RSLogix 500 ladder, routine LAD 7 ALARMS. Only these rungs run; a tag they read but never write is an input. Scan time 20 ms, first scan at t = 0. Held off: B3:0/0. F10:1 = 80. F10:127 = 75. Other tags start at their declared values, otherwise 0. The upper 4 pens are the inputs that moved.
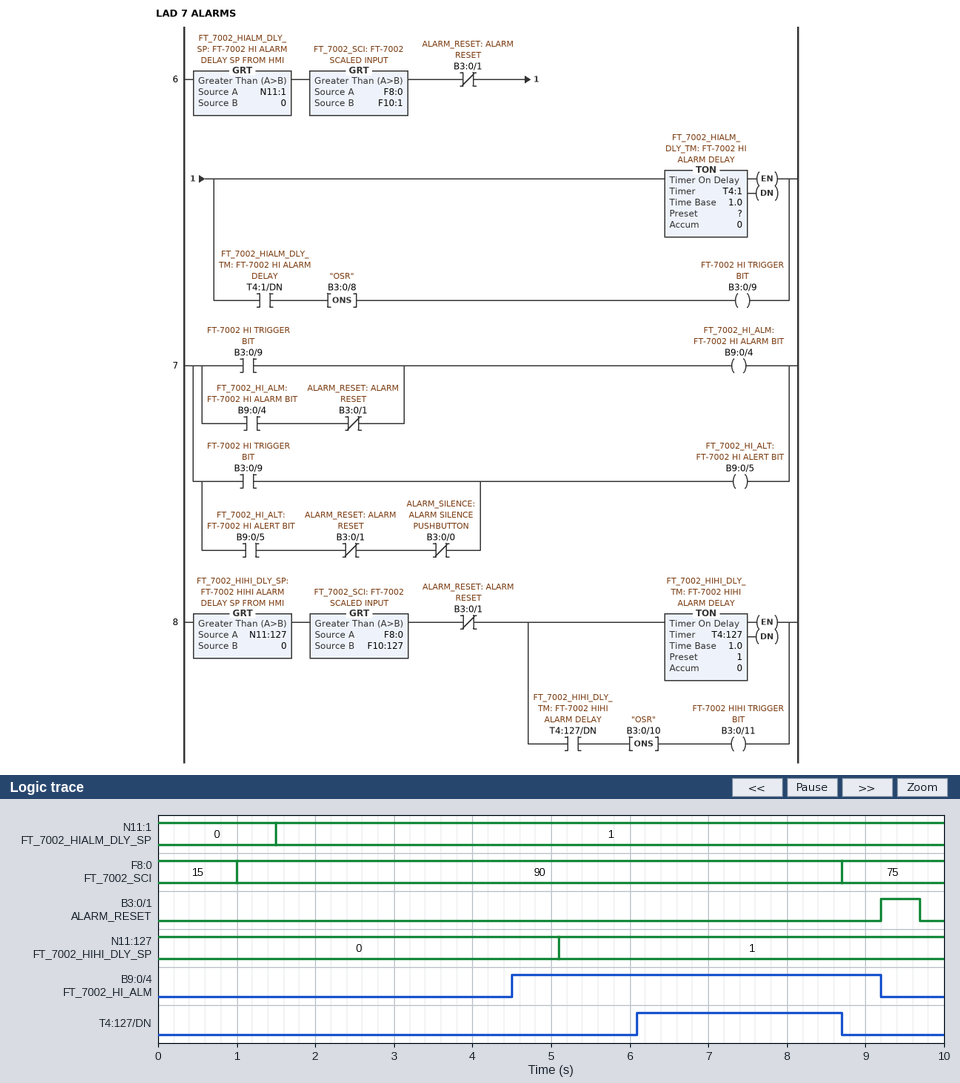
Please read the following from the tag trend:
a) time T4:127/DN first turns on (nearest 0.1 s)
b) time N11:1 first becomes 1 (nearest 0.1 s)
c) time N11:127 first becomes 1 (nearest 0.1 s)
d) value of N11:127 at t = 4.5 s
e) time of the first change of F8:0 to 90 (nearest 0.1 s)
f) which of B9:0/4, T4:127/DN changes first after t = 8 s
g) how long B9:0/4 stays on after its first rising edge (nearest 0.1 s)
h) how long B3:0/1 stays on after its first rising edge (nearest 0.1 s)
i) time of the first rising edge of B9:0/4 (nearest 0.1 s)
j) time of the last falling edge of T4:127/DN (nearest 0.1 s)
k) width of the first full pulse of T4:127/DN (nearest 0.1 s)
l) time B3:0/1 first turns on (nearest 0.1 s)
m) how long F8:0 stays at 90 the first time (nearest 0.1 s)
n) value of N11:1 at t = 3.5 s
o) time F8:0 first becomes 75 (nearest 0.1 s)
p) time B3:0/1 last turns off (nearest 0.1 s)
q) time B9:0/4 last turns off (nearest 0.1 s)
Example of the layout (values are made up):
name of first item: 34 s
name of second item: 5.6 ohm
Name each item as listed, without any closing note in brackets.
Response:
time T4:127/DN first turns on: 6.1 s
time N11:1 first becomes 1: 1.5 s
time N11:127 first becomes 1: 5.1 s
value of N11:127 at t = 4.5 s: 0
time of the first change of F8:0 to 90: 1.0 s
which of B9:0/4, T4:127/DN changes first after t = 8 s: T4:127/DN
how long B9:0/4 stays on after its first rising edge: 4.7 s
how long B3:0/1 stays on after its first rising edge: 0.5 s
time of the first rising edge of B9:0/4: 4.5 s
time of the last falling edge of T4:127/DN: 8.7 s
width of the first full pulse of T4:127/DN: 2.6 s
time B3:0/1 first turns on: 9.2 s
how long F8:0 stays at 90 the first time: 7.7 s
value of N11:1 at t = 3.5 s: 1
time F8:0 first becomes 75: 8.7 s
time B3:0/1 last turns off: 9.7 s
time B9:0/4 last turns off: 9.2 s
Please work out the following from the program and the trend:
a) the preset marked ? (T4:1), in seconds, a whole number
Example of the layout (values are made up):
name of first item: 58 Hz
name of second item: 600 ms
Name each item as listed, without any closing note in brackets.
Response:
the preset marked ? (T4:1), in seconds, a whole number: 3 s
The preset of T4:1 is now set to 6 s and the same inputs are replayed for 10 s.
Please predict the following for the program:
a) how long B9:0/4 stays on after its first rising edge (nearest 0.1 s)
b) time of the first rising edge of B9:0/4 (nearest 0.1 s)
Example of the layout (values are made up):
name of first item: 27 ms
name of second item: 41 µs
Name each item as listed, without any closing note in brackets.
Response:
how long B9:0/4 stays on after its first rising edge: 1.7 s
time of the first rising edge of B9:0/4: 7.5 s
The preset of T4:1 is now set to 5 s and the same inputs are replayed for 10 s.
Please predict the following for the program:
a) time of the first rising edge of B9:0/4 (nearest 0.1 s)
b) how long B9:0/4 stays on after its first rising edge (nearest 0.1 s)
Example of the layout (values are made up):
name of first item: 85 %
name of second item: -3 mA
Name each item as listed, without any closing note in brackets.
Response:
time of the first rising edge of B9:0/4: 6.5 s
how long B9:0/4 stays on after its first rising edge: 2.7 s
